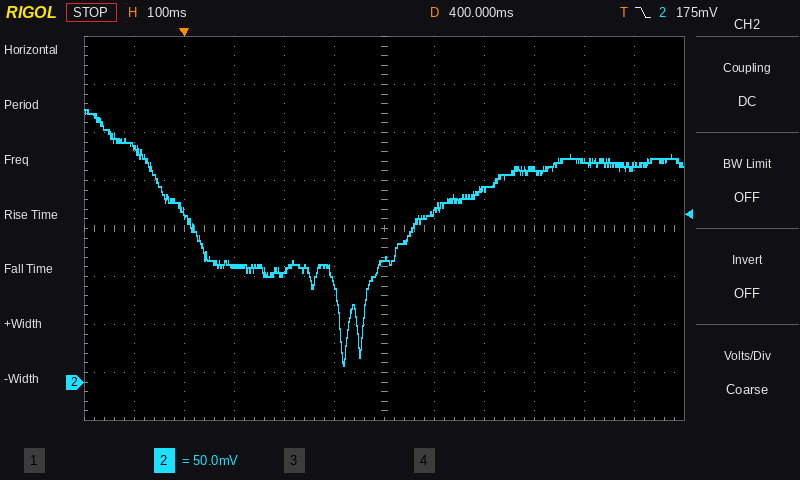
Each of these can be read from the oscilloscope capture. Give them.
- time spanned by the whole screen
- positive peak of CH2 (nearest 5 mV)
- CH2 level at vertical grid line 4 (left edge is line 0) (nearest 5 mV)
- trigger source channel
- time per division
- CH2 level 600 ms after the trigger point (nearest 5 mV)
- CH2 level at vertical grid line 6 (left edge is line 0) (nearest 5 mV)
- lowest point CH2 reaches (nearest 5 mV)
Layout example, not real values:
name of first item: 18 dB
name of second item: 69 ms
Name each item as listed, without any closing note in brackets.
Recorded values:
time spanned by the whole screen: 1.2 s
positive peak of CH2: 285 mV
CH2 level at vertical grid line 4 (left edge is line 0): 115 mV
trigger source channel: CH2
time per division: 100 ms
CH2 level 600 ms after the trigger point: 200 mV
CH2 level at vertical grid line 6 (left edge is line 0): 130 mV
lowest point CH2 reaches: 15 mV
